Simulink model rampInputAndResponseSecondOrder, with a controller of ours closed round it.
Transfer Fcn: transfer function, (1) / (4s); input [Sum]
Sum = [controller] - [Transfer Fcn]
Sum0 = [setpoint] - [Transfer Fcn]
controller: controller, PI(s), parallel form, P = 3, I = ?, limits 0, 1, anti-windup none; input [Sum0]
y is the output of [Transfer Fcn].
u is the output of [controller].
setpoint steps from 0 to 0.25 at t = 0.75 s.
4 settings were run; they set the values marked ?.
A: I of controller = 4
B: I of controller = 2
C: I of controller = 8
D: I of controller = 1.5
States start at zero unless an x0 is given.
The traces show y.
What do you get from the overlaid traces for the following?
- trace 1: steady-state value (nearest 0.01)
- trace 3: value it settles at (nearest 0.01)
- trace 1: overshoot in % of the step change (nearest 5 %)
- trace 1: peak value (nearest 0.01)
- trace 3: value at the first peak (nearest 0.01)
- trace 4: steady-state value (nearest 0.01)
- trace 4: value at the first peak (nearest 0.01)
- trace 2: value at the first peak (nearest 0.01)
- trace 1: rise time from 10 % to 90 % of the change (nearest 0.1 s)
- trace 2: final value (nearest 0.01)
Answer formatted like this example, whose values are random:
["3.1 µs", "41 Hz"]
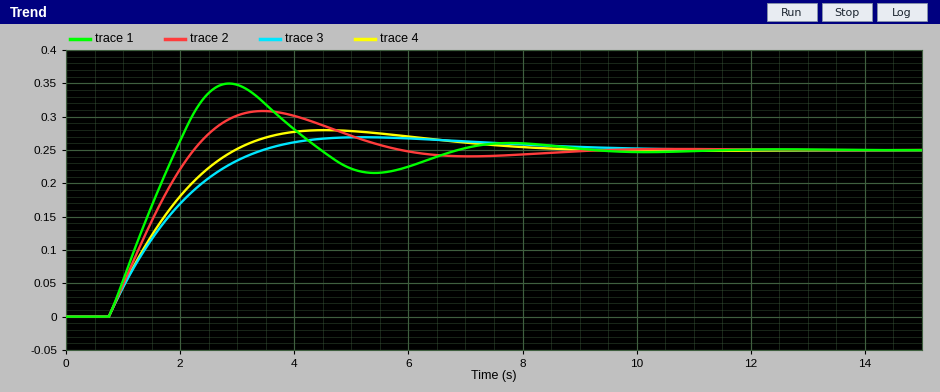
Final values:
["0.25", "0.25", "40 %", "0.35", "0.27", "0.25", "0.28", "0.31", "0.9 s", "0.25"]
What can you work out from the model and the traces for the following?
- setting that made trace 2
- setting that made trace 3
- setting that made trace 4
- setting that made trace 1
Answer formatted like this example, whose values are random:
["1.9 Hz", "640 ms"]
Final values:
["A", "D", "B", "C"]
